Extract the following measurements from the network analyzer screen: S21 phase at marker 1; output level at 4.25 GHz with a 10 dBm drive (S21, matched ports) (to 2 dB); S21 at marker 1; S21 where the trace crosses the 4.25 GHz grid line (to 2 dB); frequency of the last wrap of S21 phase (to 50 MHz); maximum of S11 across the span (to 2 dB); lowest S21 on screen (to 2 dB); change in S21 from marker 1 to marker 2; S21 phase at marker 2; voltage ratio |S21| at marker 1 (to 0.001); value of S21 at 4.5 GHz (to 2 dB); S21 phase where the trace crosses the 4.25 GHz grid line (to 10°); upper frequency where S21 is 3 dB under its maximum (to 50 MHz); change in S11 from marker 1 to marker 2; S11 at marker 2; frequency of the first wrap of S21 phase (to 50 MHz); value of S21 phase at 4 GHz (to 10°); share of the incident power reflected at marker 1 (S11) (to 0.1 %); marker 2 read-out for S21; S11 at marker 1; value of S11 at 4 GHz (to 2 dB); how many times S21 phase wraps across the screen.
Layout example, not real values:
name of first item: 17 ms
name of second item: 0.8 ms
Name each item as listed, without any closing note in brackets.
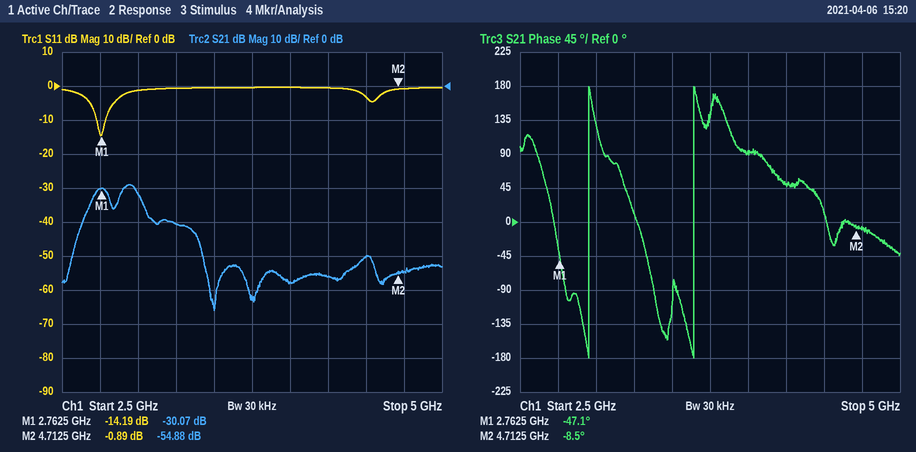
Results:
S21 phase at marker 1: -47.1°
output level at 4.25 GHz with a 10 dBm drive (S21, matched ports): -46 dBm
S21 at marker 1: -30.07 dB
S21 where the trace crosses the 4.25 GHz grid line: -56 dB
frequency of the last wrap of S21 phase: 3.65 GHz
maximum of S11 across the span: 0 dB
lowest S21 on screen: -66 dB
change in S21 from marker 1 to marker 2: -24.81 dB
S21 phase at marker 2: -8.5°
voltage ratio |S21| at marker 1: 0.031
value of S21 at 4.5 GHz: -50 dB
S21 phase where the trace crosses the 4.25 GHz grid line: 50°
upper frequency where S21 is 3 dB under its maximum: 3.00 GHz
change in S11 from marker 1 to marker 2: 13.30 dB
S11 at marker 2: -0.89 dB
frequency of the first wrap of S21 phase: 2.95 GHz
value of S21 phase at 4 GHz: 90°
share of the incident power reflected at marker 1 (S11): 3.8 %
marker 2 read-out for S21: -54.88 dB
S11 at marker 1: -14.19 dB
value of S11 at 4 GHz: 0 dB
how many times S21 phase wraps across the screen: 2
